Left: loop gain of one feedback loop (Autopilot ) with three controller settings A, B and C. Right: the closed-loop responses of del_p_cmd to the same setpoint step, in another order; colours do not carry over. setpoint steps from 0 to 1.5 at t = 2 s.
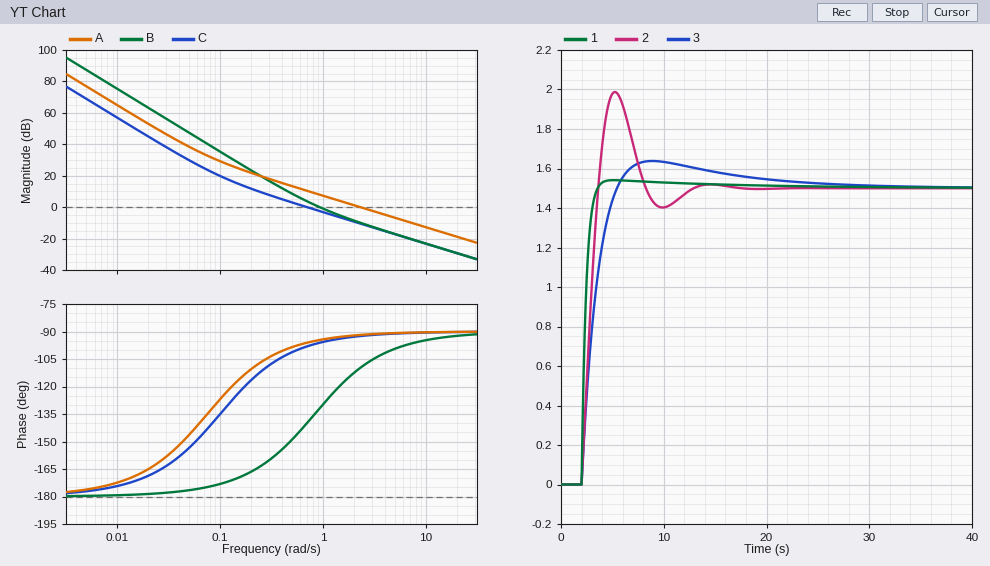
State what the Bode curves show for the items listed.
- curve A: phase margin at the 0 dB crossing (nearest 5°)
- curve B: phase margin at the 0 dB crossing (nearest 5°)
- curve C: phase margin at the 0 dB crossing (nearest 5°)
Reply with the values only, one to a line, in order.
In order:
90°
50°
80°
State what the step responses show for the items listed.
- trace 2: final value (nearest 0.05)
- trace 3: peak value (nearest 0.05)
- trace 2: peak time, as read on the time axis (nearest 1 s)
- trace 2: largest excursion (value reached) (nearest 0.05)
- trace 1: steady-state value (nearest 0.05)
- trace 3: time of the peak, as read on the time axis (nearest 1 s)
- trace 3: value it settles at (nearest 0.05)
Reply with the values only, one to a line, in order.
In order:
1.50
1.65
5 s
2.00
1.50
9 s
1.50
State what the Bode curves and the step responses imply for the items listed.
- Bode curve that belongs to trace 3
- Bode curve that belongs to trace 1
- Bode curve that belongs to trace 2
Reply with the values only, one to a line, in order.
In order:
C
A
B
